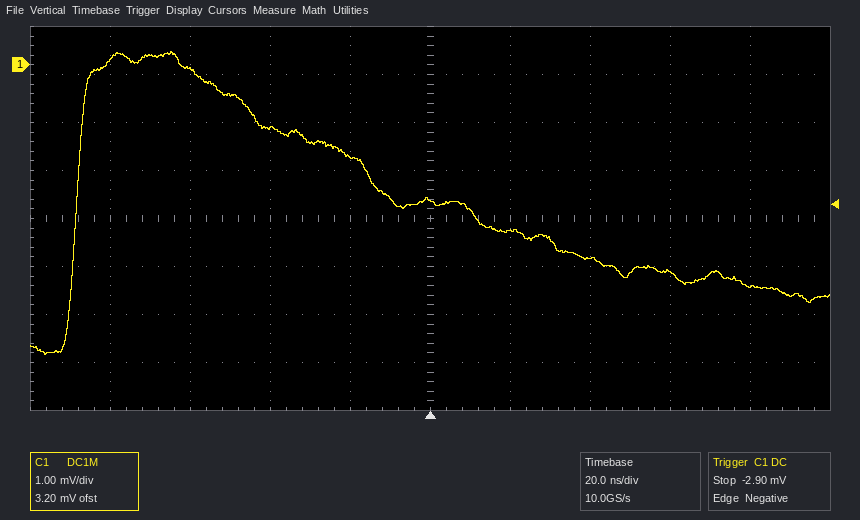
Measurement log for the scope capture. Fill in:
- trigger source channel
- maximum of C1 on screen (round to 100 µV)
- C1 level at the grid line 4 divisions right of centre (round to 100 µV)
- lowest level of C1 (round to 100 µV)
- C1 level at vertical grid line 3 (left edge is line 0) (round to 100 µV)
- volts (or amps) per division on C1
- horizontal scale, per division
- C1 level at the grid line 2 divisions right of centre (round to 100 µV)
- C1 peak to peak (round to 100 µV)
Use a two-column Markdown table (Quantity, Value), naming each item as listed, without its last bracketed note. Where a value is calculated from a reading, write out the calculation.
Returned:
| Quantity | Value |
|---|---|
| trigger source channel | C1 |
| maximum of C1 on screen | 300 µV |
| C1 level at the grid line 4 divisions right of centre | -4.6 mV |
| lowest level of C1 | -6.0 mV |
| C1 level at vertical grid line 3 (left edge is line 0) | -1.3 mV |
| volts (or amps) per division on C1 | 1 mV |
| horizontal scale, per division | 20 ns |
| C1 level at the grid line 2 divisions right of centre | -4.0 mV |
| C1 peak to peak | 300 µV − (-6.0 mV) = 6.3 mV |
